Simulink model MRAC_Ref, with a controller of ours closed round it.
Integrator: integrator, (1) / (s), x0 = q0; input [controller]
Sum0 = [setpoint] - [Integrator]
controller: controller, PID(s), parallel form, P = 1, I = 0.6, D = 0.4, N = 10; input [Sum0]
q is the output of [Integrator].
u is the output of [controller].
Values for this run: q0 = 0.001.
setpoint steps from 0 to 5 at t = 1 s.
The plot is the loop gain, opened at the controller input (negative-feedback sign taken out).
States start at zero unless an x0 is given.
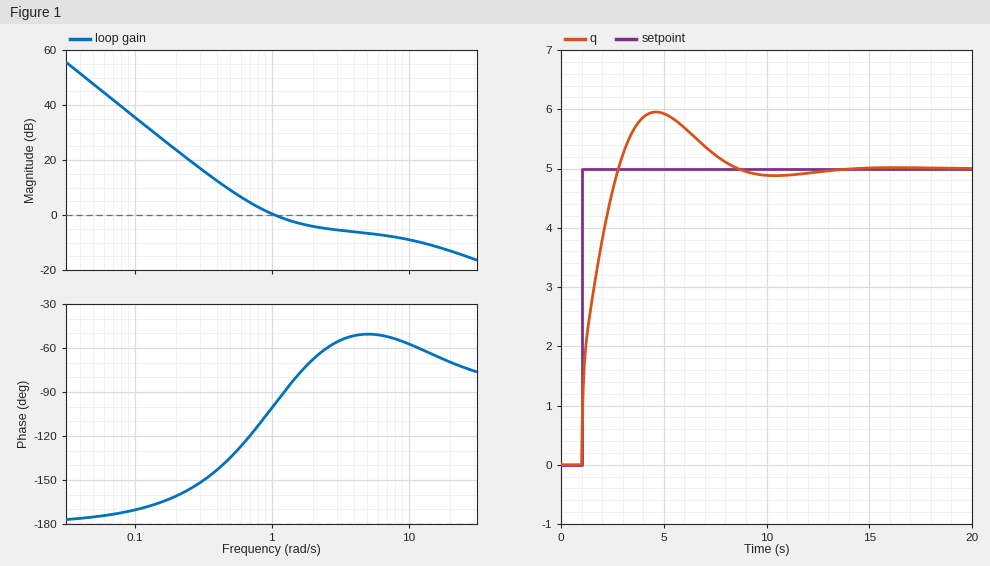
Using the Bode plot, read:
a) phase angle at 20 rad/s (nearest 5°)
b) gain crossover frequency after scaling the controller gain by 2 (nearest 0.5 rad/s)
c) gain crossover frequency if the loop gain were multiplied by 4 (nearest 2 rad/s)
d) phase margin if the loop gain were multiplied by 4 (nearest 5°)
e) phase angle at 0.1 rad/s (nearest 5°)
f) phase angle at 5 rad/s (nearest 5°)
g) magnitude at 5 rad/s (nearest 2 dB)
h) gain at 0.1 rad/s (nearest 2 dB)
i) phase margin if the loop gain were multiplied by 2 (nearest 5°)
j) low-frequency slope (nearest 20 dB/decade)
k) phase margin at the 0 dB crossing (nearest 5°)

-70°
4.0 rad/s
18 rad/s
115°
-170°
-50°
-6 dB
36 dB
130°
-40 dB/decade
80°
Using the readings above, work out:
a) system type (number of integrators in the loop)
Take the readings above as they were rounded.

2
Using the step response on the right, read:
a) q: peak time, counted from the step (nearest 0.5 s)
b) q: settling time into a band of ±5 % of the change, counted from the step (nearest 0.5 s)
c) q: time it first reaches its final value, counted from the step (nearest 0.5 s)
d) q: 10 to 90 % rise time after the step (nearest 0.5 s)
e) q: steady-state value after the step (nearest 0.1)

3.5 s
6.5 s
2.0 s
1.5 s
5.0
